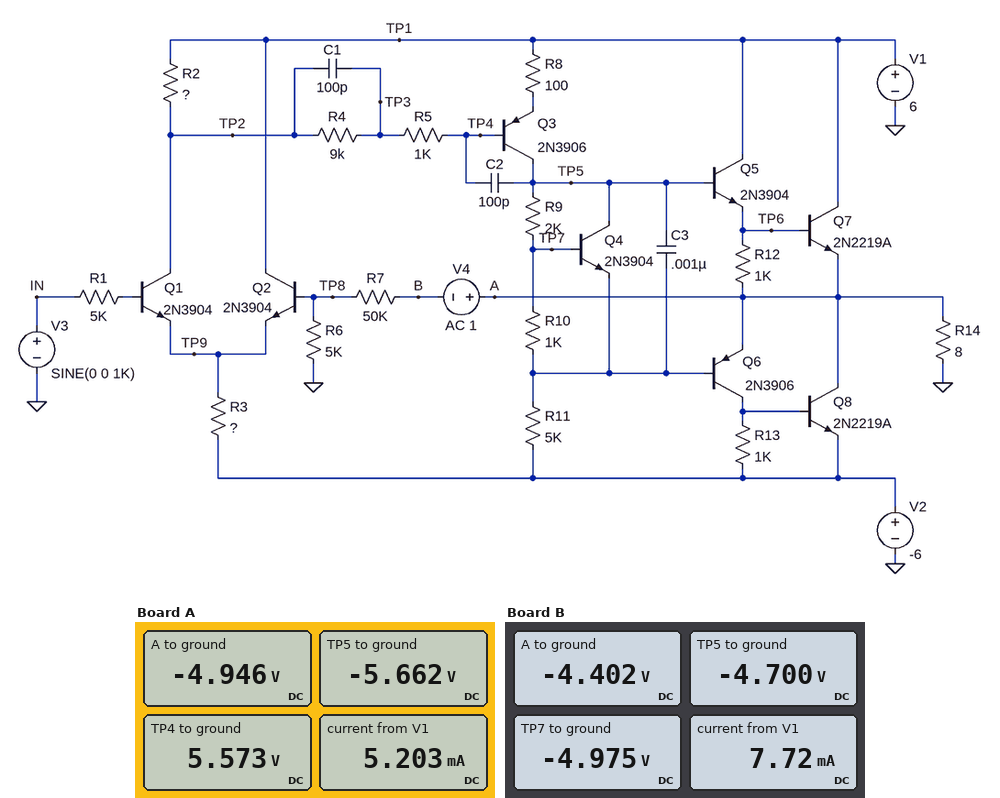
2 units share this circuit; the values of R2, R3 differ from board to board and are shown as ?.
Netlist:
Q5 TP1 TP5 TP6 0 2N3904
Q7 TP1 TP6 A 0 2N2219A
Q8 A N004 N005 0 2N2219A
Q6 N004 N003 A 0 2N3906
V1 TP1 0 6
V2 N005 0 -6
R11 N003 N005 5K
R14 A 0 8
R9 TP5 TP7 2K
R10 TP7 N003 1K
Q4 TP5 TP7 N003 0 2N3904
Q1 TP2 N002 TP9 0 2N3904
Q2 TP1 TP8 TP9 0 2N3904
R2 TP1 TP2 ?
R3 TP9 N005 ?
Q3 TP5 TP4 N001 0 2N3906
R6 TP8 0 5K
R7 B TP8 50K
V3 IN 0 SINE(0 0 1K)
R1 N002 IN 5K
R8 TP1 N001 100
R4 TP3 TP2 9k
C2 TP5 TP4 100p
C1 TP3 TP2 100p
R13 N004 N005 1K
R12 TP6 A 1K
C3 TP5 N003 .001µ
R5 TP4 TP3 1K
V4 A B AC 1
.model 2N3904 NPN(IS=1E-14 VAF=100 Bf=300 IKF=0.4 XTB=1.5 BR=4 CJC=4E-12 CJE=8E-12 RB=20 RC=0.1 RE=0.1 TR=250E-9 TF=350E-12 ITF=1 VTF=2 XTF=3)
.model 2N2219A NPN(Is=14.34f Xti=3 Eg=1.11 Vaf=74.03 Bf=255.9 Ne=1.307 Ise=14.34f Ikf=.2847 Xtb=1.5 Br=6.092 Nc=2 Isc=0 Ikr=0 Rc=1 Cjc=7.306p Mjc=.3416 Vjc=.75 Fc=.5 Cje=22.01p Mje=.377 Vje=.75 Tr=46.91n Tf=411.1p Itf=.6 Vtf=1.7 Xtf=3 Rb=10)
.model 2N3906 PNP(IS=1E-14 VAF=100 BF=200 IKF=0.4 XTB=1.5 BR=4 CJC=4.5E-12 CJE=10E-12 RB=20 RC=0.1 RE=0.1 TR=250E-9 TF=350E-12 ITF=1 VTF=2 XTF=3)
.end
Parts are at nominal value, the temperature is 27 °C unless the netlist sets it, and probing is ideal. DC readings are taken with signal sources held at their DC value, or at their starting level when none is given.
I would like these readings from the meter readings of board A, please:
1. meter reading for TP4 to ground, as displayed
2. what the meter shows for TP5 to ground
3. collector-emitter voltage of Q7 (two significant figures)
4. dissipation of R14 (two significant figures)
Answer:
5.573 V
-5.662 V
11 V
3.1 W
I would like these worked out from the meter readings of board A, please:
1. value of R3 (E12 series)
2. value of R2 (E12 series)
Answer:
1 kΩ
82 Ω
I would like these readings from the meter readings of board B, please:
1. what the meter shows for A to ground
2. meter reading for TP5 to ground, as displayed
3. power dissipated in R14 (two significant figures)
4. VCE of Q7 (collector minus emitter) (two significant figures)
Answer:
-4.402 V
-4.700 V
2.4 W
10 V
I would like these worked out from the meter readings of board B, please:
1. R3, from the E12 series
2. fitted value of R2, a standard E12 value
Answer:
680 Ω
82 Ω
